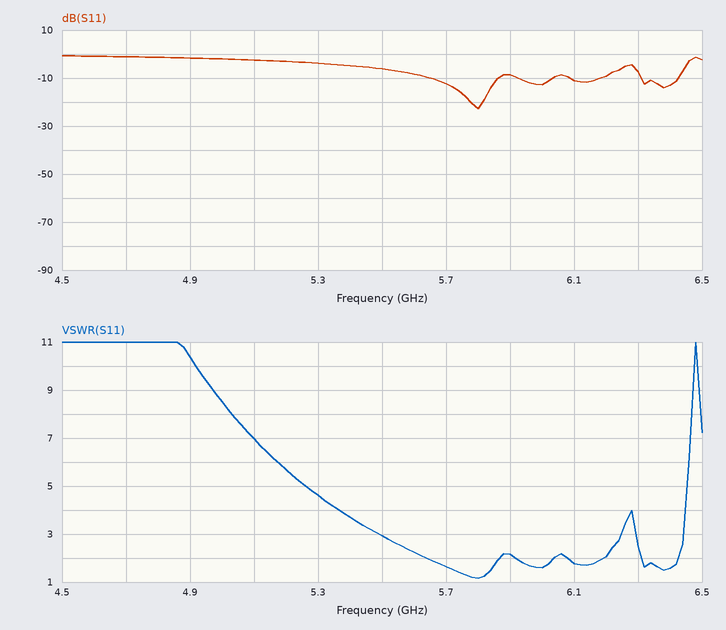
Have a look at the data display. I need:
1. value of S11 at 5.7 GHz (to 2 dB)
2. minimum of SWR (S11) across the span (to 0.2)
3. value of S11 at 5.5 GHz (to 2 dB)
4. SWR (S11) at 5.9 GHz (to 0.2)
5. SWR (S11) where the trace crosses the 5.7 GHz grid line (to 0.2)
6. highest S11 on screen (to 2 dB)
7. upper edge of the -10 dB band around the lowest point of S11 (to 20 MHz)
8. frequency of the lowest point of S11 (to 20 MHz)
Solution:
-12 dB
1.2
-6 dB
2.2
1.6
0 dB
5.86 GHz
5.80 GHz
